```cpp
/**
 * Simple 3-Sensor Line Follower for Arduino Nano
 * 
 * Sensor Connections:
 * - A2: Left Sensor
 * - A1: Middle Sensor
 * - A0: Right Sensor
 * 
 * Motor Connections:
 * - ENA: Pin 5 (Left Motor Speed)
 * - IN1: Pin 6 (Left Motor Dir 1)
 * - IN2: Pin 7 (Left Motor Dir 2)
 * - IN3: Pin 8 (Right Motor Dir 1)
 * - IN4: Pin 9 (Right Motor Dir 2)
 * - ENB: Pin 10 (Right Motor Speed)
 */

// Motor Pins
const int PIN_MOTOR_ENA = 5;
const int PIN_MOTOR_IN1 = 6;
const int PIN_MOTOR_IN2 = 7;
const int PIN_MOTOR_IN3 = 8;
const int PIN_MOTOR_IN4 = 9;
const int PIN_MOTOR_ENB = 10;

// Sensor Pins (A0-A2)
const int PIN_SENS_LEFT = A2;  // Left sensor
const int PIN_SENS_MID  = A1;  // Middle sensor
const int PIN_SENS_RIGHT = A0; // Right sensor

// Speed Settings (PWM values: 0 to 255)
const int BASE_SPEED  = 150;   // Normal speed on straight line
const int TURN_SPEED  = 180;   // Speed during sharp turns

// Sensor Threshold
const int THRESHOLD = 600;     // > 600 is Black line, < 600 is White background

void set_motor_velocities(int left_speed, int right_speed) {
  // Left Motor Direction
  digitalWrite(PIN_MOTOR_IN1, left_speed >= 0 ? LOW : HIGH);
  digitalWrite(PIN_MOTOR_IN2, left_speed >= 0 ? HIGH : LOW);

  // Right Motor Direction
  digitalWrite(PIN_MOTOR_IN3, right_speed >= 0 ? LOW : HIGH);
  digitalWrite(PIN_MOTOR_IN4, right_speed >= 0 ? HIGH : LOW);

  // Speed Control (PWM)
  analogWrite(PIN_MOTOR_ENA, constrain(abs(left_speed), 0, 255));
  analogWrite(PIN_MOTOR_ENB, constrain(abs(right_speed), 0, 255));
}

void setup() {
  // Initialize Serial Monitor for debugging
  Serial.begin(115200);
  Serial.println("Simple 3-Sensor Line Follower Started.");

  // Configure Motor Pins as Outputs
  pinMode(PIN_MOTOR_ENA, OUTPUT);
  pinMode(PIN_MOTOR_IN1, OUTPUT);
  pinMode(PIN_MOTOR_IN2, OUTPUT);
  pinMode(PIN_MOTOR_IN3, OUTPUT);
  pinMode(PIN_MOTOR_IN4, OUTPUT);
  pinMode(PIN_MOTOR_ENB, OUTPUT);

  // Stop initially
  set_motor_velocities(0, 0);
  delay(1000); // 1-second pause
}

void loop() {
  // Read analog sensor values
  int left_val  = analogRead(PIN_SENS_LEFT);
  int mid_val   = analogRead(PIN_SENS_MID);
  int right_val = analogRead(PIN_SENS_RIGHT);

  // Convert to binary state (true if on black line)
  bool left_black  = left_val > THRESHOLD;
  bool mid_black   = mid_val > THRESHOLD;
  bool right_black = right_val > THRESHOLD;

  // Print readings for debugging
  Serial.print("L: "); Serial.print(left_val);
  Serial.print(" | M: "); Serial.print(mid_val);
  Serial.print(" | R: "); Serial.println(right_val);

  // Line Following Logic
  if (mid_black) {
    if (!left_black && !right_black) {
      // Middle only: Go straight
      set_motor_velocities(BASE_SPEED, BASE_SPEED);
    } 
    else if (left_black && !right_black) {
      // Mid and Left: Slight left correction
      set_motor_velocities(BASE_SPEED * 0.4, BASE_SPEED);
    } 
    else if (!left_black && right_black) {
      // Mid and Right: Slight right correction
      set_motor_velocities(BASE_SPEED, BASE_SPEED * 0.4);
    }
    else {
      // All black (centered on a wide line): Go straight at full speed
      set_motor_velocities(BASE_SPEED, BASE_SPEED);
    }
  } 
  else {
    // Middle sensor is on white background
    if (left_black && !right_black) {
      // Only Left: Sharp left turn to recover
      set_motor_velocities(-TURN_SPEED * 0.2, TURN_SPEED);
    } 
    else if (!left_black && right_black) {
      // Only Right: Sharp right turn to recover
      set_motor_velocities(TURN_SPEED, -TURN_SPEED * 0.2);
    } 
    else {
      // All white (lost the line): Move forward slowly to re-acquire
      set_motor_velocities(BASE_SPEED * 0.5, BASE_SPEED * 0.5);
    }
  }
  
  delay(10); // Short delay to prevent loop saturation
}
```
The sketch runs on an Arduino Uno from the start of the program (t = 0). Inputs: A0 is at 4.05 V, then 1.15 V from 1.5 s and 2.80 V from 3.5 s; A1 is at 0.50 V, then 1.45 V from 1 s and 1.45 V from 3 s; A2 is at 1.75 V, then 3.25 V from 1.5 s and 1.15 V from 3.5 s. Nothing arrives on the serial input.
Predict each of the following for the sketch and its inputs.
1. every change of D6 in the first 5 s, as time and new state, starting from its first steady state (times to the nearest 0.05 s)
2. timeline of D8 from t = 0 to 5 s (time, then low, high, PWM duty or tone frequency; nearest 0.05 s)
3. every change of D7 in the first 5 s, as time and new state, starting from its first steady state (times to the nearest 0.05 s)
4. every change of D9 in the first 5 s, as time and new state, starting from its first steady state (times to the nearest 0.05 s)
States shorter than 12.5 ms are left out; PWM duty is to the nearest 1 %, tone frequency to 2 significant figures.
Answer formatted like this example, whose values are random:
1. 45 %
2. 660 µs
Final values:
1. 0 s low; 1.5 s high; 3.5 s low
2. 0 s low; 1 s high; 1.5 s low
3. 0 s high; 1.5 s low; 3.5 s high
4. 0 s high; 1 s low; 1.5 s high
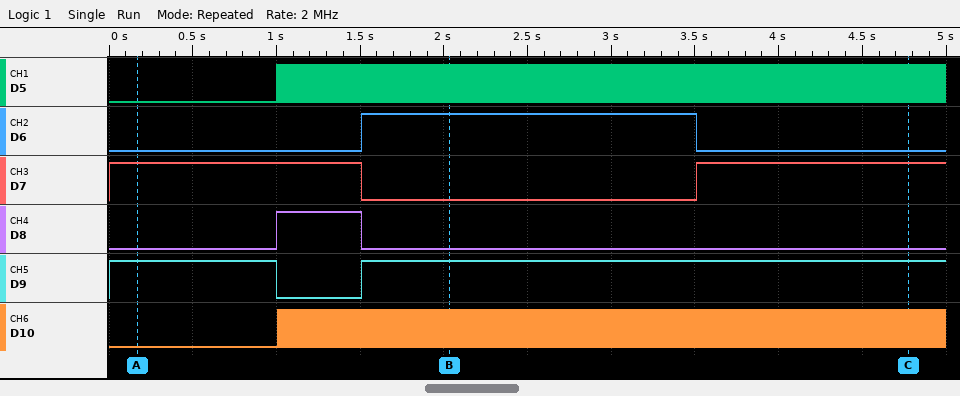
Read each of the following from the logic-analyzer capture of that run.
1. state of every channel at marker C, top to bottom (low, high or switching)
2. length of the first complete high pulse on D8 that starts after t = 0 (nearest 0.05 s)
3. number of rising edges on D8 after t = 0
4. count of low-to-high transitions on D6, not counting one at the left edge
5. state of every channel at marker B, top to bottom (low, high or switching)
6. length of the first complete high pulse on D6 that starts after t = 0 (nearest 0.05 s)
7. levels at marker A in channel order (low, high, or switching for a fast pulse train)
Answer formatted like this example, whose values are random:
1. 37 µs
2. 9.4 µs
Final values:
1. D5 switching, D6 low, D7 high, D8 low, D9 high, D10 switching
2. 0.50 s
3. 1
4. 1
5. D5 switching, D6 high, D7 low, D8 low, D9 high, D10 switching
6. 2.00 s
7. D5 low, D6 low, D7 high, D8 low, D9 high, D10 low
